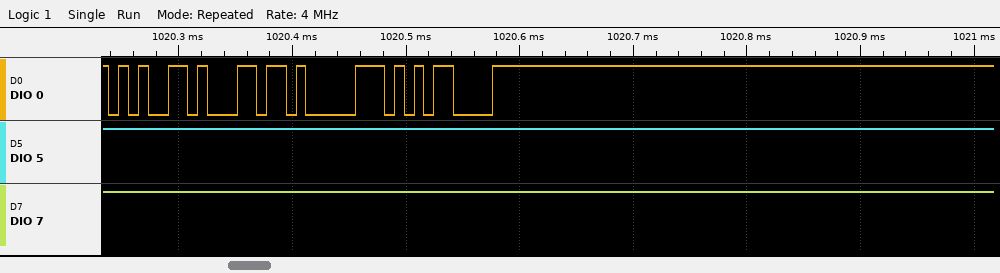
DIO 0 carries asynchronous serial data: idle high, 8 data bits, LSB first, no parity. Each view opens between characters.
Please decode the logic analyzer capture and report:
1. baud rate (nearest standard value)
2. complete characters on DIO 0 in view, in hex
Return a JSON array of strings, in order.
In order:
["115200 baud", "65, 6C, 70, 0D"]
